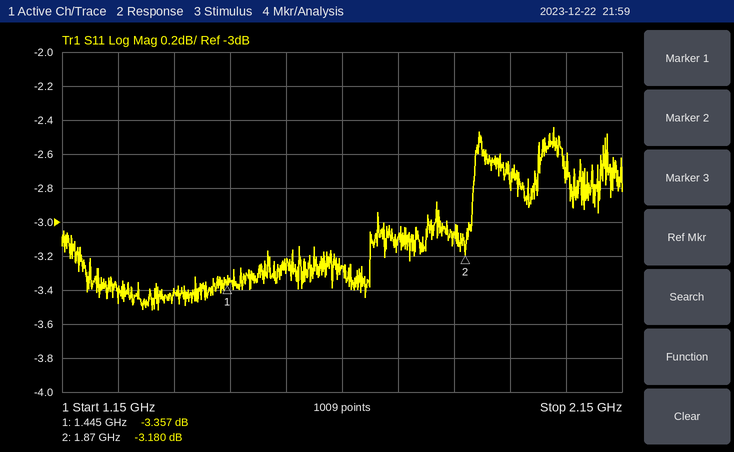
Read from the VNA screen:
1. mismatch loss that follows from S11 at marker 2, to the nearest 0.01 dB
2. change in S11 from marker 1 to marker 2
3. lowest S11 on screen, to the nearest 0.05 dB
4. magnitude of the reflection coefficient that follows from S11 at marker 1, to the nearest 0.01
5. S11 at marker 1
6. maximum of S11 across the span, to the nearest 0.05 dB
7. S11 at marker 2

2.85 dB
0.177 dB
-3.50 dB
0.68
-3.357 dB
-2.45 dB
-3.180 dB
